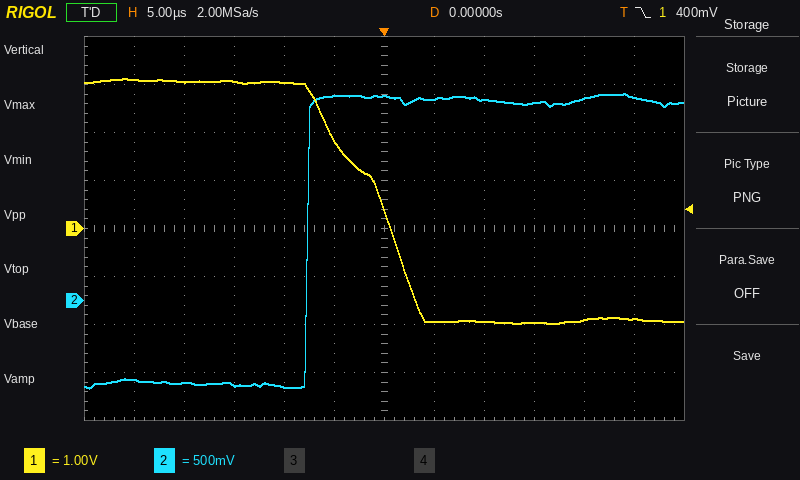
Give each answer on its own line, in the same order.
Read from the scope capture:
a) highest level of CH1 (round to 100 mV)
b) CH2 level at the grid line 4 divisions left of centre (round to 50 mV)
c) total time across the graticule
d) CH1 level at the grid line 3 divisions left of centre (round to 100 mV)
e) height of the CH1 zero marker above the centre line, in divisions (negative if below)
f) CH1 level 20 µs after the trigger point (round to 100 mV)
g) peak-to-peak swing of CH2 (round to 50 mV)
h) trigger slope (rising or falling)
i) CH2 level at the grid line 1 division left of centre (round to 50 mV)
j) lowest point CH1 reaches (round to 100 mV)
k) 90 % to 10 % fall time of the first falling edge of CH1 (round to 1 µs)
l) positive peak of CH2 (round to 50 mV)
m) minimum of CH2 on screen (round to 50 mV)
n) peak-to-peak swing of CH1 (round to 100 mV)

3.1 V
-850 mV
60 µs
3.1 V
0.0 div
-1.9 V
3.05 V
falling
2.15 V
-2.0 V
10 µs
2.15 V
-900 mV
5.1 V
